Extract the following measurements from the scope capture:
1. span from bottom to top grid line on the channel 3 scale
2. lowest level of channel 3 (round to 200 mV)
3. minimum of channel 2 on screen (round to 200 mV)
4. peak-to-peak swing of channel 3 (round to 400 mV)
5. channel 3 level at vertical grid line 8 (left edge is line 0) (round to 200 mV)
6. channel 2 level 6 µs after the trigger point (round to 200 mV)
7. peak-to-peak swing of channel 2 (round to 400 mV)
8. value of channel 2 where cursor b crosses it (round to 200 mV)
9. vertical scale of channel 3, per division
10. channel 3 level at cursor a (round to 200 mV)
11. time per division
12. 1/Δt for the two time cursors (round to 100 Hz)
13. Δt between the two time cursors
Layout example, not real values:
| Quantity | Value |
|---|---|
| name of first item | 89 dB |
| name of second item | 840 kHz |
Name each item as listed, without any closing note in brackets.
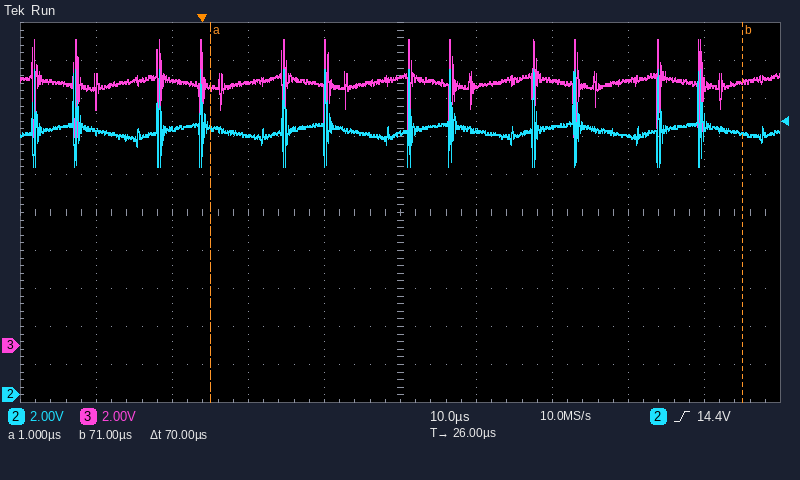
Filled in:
| Quantity | Value |
|---|---|
| span from bottom to top grid line on the channel 3 scale | 20 V |
| lowest level of channel 3 | 11.0 V |
| minimum of channel 2 on screen | 12.0 V |
| peak-to-peak swing of channel 3 | 5.2 V |
| channel 3 level at vertical grid line 8 (left edge is line 0) | 14.0 V |
| channel 2 level 6 µs after the trigger point | 13.6 V |
| peak-to-peak swing of channel 2 | 5.2 V |
| value of channel 2 where cursor b crosses it | 13.8 V |
| vertical scale of channel 3, per division | 2 V |
| channel 3 level at cursor a | 13.6 V |
| time per division | 10 µs |
| 1/Δt for the two time cursors | 14.3 kHz |
| Δt between the two time cursors | 70 µs |
